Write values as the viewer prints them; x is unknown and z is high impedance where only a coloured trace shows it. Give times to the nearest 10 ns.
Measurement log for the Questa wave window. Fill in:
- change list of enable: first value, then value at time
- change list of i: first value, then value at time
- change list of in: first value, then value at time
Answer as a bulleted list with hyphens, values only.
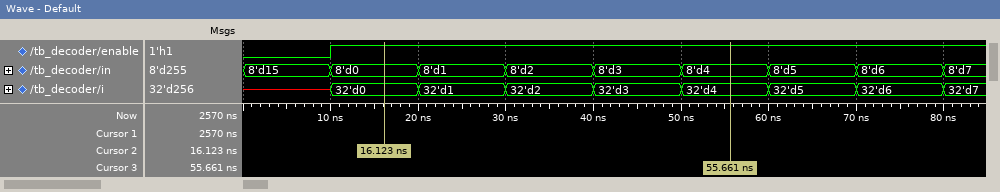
- 0, 1 at 10 ns
- x, 32'd0 at 10 ns, 32'd1 at 20 ns, 32'd2 at 30 ns, 32'd3 at 40 ns, 32'd4 at 50 ns, 32'd5 at 60 ns, 32'd6 at 70 ns, 32'd7 at 80 ns
- 8'd15, 8'd0 at 10 ns, 8'd1 at 20 ns, 8'd2 at 30 ns, 8'd3 at 40 ns, 8'd4 at 50 ns, 8'd5 at 60 ns, 8'd6 at 70 ns, 8'd7 at 80 ns
